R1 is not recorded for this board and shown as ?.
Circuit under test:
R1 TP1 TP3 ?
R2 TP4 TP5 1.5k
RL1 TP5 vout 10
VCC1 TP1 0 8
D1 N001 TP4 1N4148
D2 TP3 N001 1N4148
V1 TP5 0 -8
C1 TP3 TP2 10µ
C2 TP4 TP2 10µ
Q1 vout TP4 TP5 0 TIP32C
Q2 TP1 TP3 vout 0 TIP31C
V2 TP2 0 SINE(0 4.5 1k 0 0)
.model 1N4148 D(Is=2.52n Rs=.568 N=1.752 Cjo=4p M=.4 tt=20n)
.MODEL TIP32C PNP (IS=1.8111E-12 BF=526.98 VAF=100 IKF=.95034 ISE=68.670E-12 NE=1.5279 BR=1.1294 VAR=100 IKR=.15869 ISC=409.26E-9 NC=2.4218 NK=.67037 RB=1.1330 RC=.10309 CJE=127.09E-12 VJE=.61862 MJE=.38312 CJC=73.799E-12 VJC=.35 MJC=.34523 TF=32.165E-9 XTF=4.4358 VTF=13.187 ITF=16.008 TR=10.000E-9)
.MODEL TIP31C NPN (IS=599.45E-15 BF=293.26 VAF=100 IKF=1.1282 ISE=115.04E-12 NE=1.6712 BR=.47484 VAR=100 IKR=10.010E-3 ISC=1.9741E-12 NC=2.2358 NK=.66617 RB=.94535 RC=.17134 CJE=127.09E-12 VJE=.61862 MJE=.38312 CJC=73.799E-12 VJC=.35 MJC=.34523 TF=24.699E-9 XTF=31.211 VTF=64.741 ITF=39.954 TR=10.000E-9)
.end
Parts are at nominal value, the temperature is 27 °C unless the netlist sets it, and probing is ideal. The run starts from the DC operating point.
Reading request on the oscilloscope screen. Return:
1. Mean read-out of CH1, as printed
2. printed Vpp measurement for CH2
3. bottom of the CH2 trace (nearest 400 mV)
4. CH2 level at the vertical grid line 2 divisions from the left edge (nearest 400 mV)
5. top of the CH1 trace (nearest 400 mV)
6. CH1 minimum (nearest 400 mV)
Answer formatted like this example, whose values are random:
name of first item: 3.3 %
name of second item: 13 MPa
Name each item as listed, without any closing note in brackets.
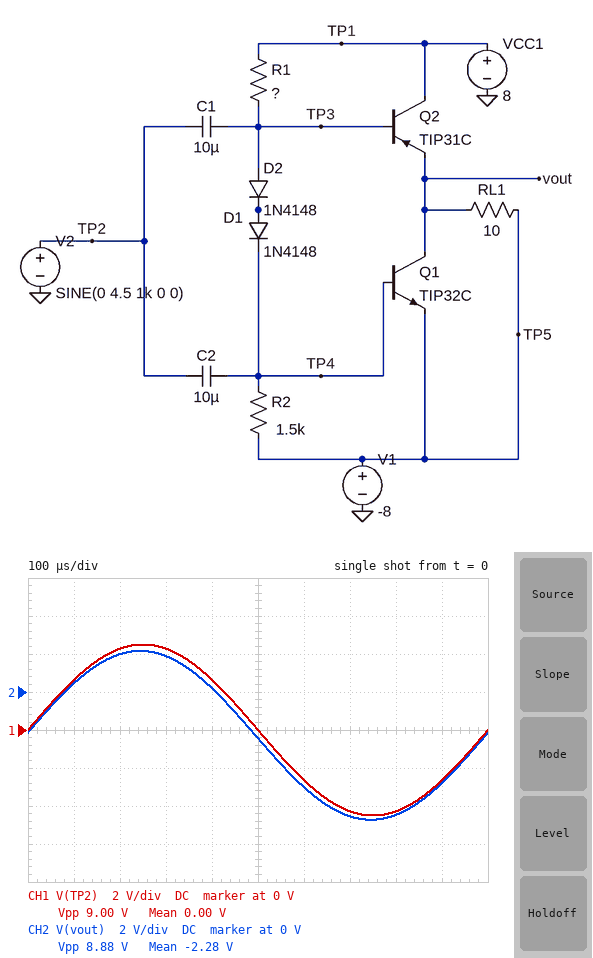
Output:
Mean read-out of CH1, as printed: 0.00 V
printed Vpp measurement for CH2: 8.88 V
bottom of the CH2 trace: -6.8 V
CH2 level at the vertical grid line 2 divisions from the left edge: 2.0 V
top of the CH1 trace: 4.4 V
CH1 minimum: -4.4 V
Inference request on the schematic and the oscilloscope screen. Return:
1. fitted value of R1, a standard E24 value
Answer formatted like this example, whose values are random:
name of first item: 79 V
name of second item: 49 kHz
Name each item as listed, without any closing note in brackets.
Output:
fitted value of R1, a standard E24 value: 1.2 kΩ
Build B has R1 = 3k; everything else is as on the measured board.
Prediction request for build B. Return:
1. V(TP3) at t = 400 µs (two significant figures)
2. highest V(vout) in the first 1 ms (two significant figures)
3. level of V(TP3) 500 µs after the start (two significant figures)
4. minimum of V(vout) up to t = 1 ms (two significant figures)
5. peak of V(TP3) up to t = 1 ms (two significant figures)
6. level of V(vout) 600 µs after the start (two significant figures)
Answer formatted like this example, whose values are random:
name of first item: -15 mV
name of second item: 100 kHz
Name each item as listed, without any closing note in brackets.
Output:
V(TP3) at t = 400 µs: -1.5 V
highest V(vout) in the first 1 ms: -290 mV
level of V(TP3) 500 µs after the start: -4.1 V
minimum of V(vout) up to t = 1 ms: -8.0 V
peak of V(TP3) up to t = 1 ms: 460 mV
level of V(vout) 600 µs after the start: -7.4 V
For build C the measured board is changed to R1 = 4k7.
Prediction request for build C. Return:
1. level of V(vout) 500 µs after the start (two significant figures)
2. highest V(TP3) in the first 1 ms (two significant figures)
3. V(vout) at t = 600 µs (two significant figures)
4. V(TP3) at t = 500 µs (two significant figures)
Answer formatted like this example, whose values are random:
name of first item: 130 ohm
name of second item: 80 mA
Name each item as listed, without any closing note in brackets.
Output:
level of V(vout) 500 µs after the start: -5.8 V
highest V(TP3) in the first 1 ms: -510 mV
V(vout) at t = 600 µs: -8.0 V
V(TP3) at t = 500 µs: -5.1 V
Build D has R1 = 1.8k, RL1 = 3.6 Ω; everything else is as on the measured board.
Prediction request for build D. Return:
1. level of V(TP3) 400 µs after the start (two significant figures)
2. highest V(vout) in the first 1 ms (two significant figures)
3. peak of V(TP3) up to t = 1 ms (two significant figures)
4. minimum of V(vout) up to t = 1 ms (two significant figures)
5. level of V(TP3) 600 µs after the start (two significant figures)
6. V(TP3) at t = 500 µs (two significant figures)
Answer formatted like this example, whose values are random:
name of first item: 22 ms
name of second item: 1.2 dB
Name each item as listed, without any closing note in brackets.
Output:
level of V(TP3) 400 µs after the start: -3.1 V
highest V(vout) in the first 1 ms: -1.7 V
peak of V(TP3) up to t = 1 ms: -920 mV
minimum of V(vout) up to t = 1 ms: -8.0 V
level of V(TP3) 600 µs after the start: -8.4 V
V(TP3) at t = 500 µs: -5.8 V
